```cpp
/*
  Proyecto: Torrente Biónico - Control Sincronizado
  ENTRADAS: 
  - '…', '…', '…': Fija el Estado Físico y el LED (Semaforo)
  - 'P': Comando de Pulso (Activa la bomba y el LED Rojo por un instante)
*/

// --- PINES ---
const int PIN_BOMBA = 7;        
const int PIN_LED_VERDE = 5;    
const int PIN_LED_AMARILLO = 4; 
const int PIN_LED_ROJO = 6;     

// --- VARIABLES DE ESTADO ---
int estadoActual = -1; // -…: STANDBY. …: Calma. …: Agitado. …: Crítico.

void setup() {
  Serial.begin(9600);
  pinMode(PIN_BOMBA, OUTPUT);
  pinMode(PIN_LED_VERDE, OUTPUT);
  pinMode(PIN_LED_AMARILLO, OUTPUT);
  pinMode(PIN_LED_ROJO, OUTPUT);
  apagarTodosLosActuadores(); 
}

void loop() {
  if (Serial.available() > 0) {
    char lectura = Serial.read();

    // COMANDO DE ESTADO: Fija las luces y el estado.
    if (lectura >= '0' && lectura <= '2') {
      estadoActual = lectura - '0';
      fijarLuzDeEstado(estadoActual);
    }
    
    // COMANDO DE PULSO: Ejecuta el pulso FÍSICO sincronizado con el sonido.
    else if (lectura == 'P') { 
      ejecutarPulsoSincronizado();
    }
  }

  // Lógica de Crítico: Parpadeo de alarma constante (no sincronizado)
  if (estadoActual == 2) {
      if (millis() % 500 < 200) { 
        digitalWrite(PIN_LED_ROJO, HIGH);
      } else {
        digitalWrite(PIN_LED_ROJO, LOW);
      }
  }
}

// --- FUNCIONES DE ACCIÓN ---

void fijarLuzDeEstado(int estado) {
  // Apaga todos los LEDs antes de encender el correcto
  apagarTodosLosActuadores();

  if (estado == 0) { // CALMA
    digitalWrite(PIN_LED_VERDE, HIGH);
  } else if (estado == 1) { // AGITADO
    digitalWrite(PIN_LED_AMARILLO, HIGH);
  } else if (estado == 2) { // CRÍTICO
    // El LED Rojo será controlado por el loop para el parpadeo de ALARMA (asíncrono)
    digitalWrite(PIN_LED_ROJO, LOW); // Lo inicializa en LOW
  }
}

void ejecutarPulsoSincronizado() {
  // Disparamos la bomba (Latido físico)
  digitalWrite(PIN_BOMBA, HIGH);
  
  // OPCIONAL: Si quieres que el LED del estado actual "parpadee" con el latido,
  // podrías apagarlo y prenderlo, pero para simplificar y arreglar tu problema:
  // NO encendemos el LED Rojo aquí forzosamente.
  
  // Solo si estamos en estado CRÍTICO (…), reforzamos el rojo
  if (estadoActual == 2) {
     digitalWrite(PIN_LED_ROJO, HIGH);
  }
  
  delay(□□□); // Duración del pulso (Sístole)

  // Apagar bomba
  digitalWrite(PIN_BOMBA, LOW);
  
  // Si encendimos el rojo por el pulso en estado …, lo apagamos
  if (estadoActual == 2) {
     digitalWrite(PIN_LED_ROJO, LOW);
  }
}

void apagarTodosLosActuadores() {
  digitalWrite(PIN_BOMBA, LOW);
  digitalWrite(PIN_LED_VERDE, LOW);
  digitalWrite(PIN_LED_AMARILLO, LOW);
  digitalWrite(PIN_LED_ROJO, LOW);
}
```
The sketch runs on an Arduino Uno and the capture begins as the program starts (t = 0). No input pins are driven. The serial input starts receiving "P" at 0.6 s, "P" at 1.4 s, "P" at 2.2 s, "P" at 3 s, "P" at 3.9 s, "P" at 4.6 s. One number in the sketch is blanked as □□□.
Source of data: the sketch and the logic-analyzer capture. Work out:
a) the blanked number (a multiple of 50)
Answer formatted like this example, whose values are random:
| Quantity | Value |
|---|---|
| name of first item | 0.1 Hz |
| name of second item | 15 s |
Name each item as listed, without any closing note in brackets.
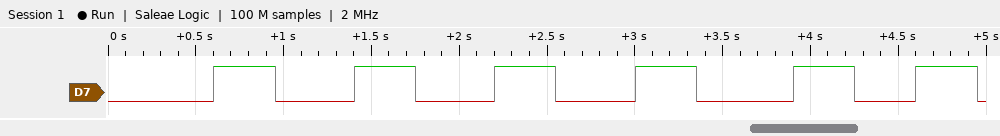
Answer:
| Quantity | Value |
|---|---|
| the blanked number | 350 |
